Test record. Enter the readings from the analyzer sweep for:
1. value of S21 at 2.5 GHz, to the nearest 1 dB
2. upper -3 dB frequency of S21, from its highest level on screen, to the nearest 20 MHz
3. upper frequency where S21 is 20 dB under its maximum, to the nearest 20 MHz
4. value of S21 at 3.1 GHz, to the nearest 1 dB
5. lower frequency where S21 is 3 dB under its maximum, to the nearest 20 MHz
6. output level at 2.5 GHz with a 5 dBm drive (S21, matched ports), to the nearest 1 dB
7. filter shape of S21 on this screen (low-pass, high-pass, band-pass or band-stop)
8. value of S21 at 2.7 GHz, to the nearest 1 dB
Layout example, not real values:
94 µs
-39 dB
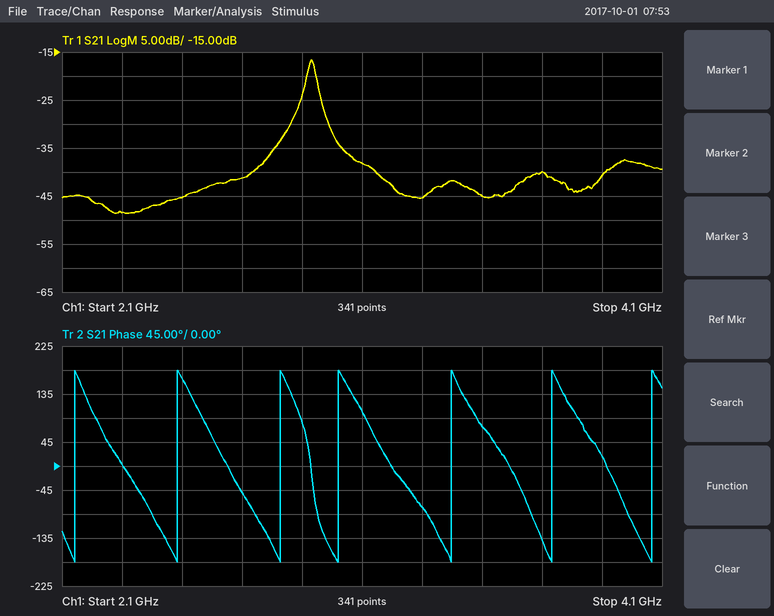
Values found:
-45 dB
2.94 GHz
3.06 GHz
-38 dB
2.92 GHz
-40 dBm
band-pass
-41 dB
